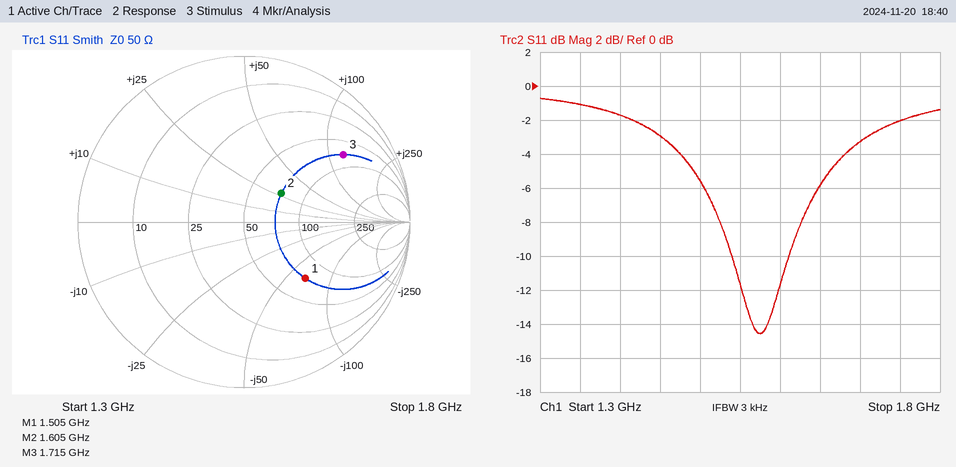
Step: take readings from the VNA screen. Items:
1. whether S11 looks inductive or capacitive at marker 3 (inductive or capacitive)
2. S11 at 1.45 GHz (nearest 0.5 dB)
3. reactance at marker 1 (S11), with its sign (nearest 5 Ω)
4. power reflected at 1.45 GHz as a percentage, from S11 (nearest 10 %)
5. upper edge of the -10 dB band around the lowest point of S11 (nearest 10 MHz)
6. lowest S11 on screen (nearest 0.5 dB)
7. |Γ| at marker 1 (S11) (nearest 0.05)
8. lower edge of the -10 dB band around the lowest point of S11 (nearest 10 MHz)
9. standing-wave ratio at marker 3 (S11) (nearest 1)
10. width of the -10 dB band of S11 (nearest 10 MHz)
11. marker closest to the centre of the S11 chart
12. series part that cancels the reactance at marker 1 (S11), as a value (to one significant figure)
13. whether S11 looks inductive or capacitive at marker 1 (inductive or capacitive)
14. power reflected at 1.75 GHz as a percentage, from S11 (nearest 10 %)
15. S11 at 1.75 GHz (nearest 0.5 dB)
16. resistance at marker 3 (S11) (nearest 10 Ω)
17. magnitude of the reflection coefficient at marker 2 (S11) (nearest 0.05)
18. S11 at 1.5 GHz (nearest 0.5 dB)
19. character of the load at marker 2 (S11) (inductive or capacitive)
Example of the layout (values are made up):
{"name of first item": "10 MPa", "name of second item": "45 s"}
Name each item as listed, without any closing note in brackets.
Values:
{"whether S11 looks inductive or capacitive at marker 3": "inductive", "S11 at 1.45 GHz": "-3.0 dB", "reactance at marker 1 (S11), with its sign": "-65 Ω", "power reflected at 1.45 GHz as a percentage, from S11": "50 %", "upper edge of the -10 dB band around the lowest point of S11": "1.61 GHz", "lowest S11 on screen": "-14.5 dB", "|Γ| at marker 1 (S11)": "0.50", "lower edge of the -10 dB band around the lowest point of S11": "1.54 GHz", "standing-wave ratio at marker 3 (S11)": "6", "width of the -10 dB band of S11": "70 MHz", "marker closest to the centre of the S11 chart": "marker 2", "series part that cancels the reactance at marker 1 (S11), as a value": "7 nH", "whether S11 looks inductive or capacitive at marker 1": "capacitive", "power reflected at 1.75 GHz as a percentage, from S11": "60 %", "S11 at 1.75 GHz": "-2.0 dB", "resistance at marker 3 (S11)": "70 Ω", "magnitude of the reflection coefficient at marker 2 (S11)": "0.30", "S11 at 1.5 GHz": "-5.5 dB", "character of the load at marker 2 (S11)": "inductive"}
